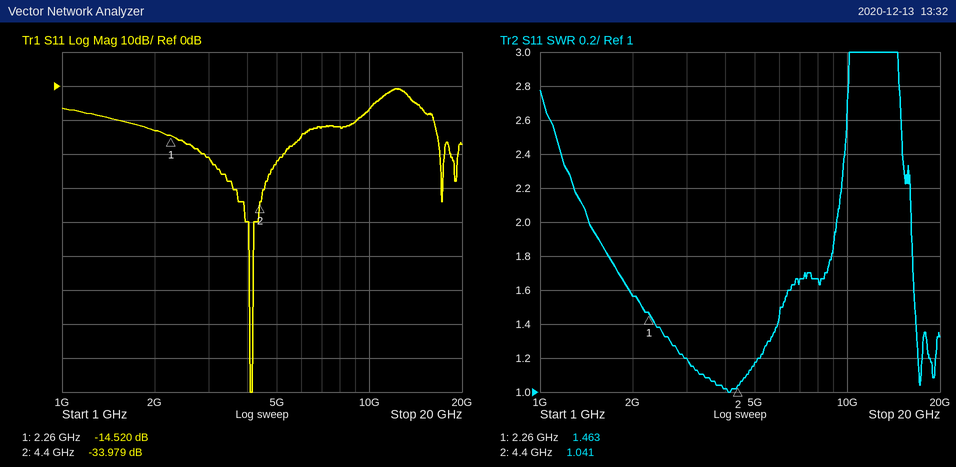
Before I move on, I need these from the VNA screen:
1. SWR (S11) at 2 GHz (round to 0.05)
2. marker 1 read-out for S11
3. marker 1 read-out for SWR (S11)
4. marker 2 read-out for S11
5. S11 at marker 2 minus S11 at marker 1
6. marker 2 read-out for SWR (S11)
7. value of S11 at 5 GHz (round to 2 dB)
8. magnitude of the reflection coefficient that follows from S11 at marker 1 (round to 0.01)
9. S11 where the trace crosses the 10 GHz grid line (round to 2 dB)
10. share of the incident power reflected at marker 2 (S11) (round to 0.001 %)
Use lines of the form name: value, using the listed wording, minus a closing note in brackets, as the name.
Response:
SWR (S11) at 2 GHz: 1.55
marker 1 read-out for S11: -14.520 dB
marker 1 read-out for SWR: 1.463
marker 2 read-out for S11: -33.979 dB
S11 at marker 2 minus S11 at marker 1: -19.459 dB
marker 2 read-out for SWR: 1.041
value of S11 at 5 GHz: -22 dB
magnitude of the reflection coefficient that follows from S11 at marker 1: 0.19
S11 where the trace crosses the 10 GHz grid line: -6 dB
share of the incident power reflected at marker 2 (S11): 0.040 %
